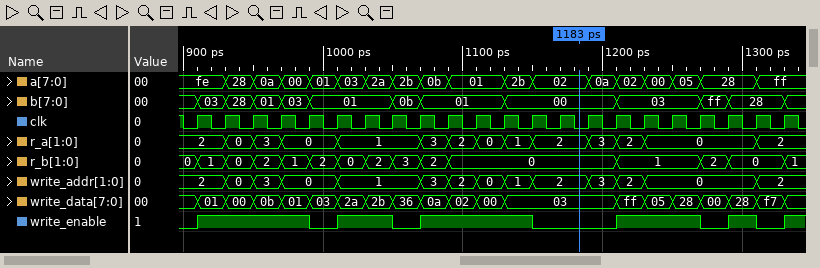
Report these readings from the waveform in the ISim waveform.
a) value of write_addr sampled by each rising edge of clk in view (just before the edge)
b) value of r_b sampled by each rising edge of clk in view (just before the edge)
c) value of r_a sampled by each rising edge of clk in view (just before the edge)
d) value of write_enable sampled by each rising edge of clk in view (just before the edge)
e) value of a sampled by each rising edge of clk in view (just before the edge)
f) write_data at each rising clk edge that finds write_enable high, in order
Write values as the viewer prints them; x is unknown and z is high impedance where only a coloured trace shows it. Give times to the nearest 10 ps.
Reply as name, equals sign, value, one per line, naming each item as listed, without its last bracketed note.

value of write_addr sampled by each rising edge of clk in view = 2, 2, 0, 3, 0, 0, 1, 1, 1, 3, 2, 0, 1, 2, 2, 3, 2, 0, 0, 0, 0, 2
value of r_b sampled by each rising edge of clk in view = 0, 1, 0, 2, 1, 2, 0, 2, 3, 2, 0, 0, 0, 0, 0, 0, 1, 1, 1, 2, 0, 0
value of r_a sampled by each rising edge of clk in view = 2, 2, 0, 3, 0, 0, 1, 1, 1, 3, 2, 0, 1, 2, 2, 3, 2, 0, 0, 0, 0, 2
value of write_enable sampled by each rising edge of clk in view = 0 1 1 1 1 0 1 1 0 1 1 1 1 0 0 0 1 1 1 0 1 0
value of a sampled by each rising edge of clk in view = fe, fe, 28, 0a, 00, 01, 03, 2a, 2b, 0b, 01, 01, 2b, 02, 02, 0a, 02, 00, 05, 28, 28, ff
write_data at each rising clk edge that finds write_enable high, in order = 01, 00, 0b, 01, 2a, 2b, 0a, 02, 00, 03, ff, 05, 28, 28
